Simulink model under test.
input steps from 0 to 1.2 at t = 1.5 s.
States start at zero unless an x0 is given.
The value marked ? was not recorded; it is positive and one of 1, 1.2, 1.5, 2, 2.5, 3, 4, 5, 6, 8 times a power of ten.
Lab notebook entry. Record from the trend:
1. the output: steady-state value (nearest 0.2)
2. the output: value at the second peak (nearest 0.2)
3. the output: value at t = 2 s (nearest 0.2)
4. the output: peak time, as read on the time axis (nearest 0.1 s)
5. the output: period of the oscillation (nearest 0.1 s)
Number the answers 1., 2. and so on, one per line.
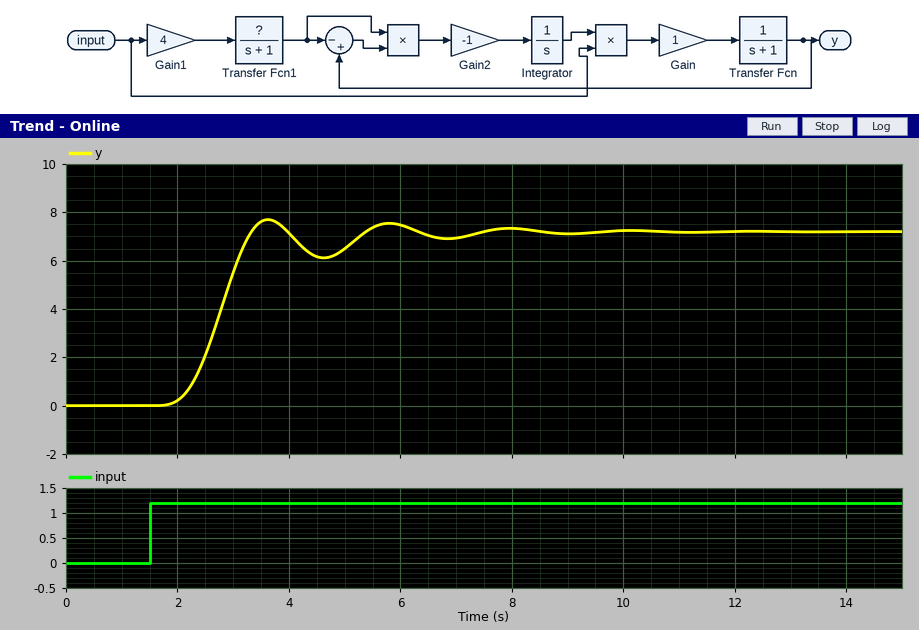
1. 7.2
2. 7.6
3. 0.2
4. 3.6 s
5. 2.2 s
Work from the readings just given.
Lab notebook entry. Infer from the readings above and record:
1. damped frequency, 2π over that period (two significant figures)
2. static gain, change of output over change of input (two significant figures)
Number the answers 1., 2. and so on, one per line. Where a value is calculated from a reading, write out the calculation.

1. 2π / 2.2 = 2.9 rad/s
2. (7.2 - 0) / (1.2 - 0) = 6.0
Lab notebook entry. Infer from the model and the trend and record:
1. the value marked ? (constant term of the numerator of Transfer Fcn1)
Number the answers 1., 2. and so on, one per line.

1. 1.5
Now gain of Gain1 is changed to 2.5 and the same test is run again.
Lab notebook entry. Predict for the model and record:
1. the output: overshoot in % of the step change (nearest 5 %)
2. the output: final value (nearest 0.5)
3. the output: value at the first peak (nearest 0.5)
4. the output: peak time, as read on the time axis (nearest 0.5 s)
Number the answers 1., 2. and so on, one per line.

1. 10 %
2. 4.5
3. 5.0
4. 4.0 s
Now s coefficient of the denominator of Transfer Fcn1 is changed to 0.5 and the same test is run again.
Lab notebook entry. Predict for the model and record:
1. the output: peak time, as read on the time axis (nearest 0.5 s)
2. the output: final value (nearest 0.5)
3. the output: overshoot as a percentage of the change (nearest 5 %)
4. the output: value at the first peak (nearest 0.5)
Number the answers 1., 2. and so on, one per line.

1. 3.0 s
2. 7.0
3. 30 %
4. 9.5
